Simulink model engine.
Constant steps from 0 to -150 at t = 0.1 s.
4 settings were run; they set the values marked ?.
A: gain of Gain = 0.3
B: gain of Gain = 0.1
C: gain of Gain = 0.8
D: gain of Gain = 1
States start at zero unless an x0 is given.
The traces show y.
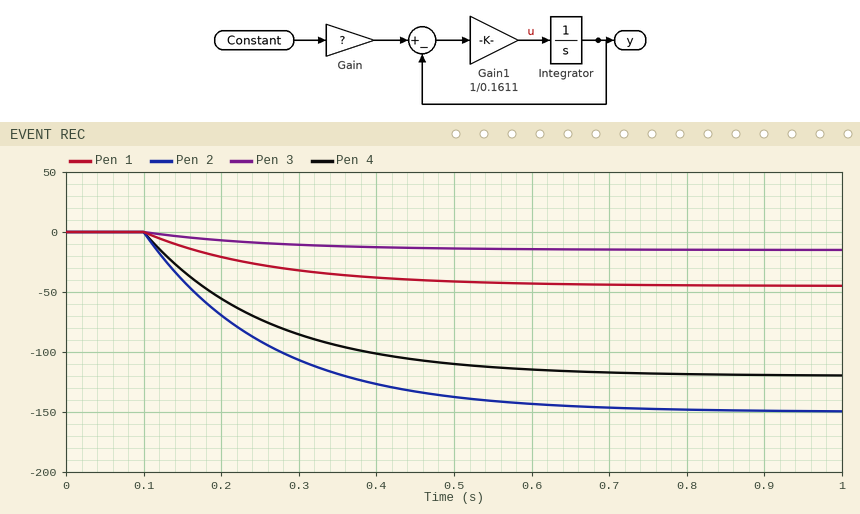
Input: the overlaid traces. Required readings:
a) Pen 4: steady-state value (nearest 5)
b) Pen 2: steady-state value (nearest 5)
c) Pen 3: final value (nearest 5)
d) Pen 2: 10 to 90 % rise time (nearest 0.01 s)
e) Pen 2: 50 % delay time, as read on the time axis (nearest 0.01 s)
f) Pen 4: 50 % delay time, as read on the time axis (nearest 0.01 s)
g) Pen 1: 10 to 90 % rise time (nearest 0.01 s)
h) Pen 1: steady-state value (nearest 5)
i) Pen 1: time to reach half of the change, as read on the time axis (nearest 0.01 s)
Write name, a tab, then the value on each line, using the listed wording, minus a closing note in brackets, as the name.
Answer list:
Pen 4: steady-state value	-120
Pen 2: steady-state value	-150
Pen 3: final value	-15
Pen 2: 10 to 90 % rise time	0.35 s
Pen 2: 50 % delay time, as read on the time axis	0.21 s
Pen 4: 50 % delay time, as read on the time axis	0.21 s
Pen 1: 10 to 90 % rise time	0.35 s
Pen 1: steady-state value	-45
Pen 1: time to reach half of the change, as read on the time axis	0.21 s
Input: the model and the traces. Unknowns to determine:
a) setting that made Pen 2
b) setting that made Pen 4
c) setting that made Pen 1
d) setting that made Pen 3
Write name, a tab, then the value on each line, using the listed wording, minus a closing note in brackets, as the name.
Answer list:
setting that made Pen 2	D
setting that made Pen 4	C
setting that made Pen 1	A
setting that made Pen 3	B
